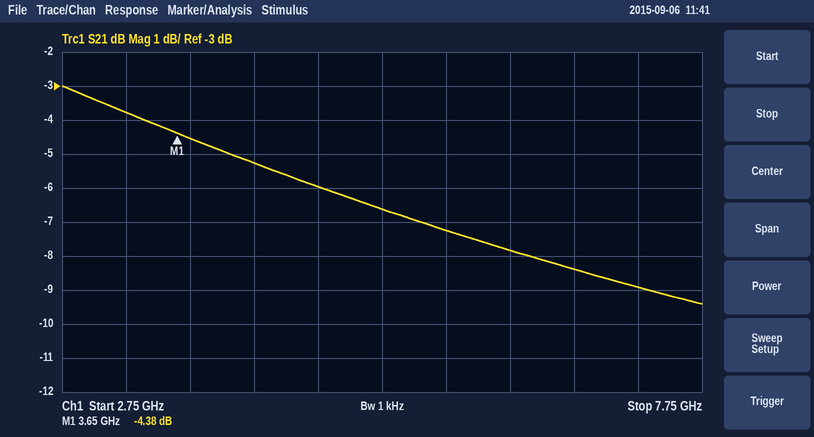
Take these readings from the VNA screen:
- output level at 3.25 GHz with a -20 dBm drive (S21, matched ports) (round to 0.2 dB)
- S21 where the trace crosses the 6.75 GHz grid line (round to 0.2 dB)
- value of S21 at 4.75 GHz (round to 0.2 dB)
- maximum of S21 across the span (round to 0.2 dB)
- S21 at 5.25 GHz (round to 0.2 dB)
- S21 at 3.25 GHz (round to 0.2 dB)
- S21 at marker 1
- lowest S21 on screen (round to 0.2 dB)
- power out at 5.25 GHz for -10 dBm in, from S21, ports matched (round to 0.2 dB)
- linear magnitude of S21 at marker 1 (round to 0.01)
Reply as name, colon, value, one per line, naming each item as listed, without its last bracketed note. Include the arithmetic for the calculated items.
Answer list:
output level at 3.25 GHz with a -20 dBm drive (S21, matched ports): -20 dBm + (-3.8 dB) = -23.8 dBm
S21 where the trace crosses the 6.75 GHz grid line: -8.4 dB
value of S21 at 4.75 GHz: -6.0 dB
maximum of S21 across the span: -3.0 dB
S21 at 5.25 GHz: -6.6 dB
S21 at 3.25 GHz: -3.8 dB
S21 at marker 1: -4.38 dB
lowest S21 on screen: -9.4 dB
power out at 5.25 GHz for -10 dBm in, from S21, ports matched: -10 dBm + (-6.6 dB) = -16.6 dBm
linear magnitude of S21 at marker 1: 10^(-4.38/20) ≈ 0.60
